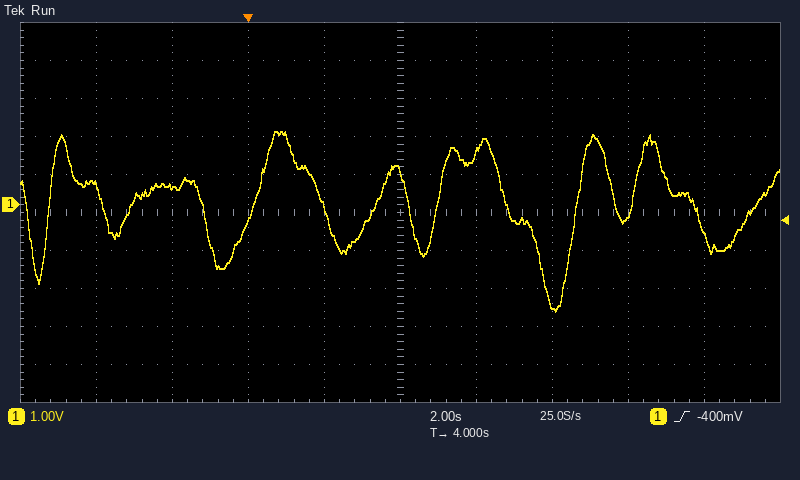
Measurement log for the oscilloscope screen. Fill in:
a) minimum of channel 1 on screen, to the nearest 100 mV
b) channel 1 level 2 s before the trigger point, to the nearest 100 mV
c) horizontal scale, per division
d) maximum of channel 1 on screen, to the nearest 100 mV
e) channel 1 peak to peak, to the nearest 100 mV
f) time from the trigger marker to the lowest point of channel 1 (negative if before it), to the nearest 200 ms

-2.8 V
500 mV
2 s
1.9 V
4.7 V
+8.0 s
